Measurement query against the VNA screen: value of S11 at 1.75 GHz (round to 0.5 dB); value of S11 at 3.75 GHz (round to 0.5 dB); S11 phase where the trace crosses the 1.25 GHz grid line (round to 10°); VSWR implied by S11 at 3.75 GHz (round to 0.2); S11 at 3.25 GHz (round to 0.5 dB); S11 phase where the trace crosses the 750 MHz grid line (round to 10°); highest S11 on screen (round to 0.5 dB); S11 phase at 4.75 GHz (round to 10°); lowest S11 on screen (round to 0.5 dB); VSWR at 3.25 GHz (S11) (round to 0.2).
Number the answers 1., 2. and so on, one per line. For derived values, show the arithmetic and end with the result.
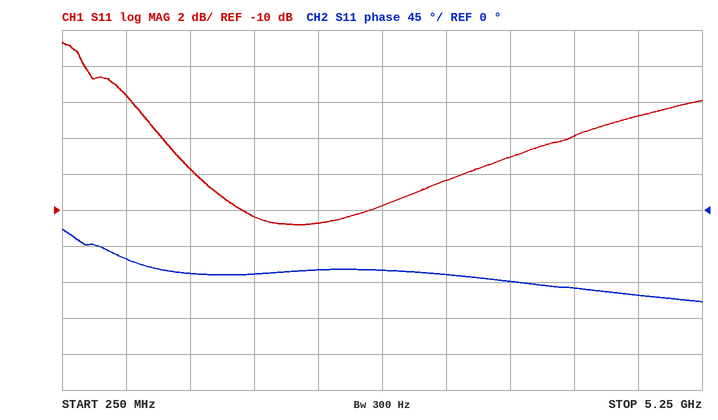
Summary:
1. -10.5 dB
2. -7.0 dB
3. -80°
4. |Γ| = 10^(-7/20) = 0.4467; VSWR = (1 + 0.4467)/(1 − 0.4467) ≈ 2.6
5. -8.5 dB
6. -60°
7. -0.5 dB
8. -110°
9. -11.0 dB
10. |Γ| = 10^(-8.5/20) = 0.3758; VSWR = (1 + 0.3758)/(1 − 0.3758) ≈ 2.2
